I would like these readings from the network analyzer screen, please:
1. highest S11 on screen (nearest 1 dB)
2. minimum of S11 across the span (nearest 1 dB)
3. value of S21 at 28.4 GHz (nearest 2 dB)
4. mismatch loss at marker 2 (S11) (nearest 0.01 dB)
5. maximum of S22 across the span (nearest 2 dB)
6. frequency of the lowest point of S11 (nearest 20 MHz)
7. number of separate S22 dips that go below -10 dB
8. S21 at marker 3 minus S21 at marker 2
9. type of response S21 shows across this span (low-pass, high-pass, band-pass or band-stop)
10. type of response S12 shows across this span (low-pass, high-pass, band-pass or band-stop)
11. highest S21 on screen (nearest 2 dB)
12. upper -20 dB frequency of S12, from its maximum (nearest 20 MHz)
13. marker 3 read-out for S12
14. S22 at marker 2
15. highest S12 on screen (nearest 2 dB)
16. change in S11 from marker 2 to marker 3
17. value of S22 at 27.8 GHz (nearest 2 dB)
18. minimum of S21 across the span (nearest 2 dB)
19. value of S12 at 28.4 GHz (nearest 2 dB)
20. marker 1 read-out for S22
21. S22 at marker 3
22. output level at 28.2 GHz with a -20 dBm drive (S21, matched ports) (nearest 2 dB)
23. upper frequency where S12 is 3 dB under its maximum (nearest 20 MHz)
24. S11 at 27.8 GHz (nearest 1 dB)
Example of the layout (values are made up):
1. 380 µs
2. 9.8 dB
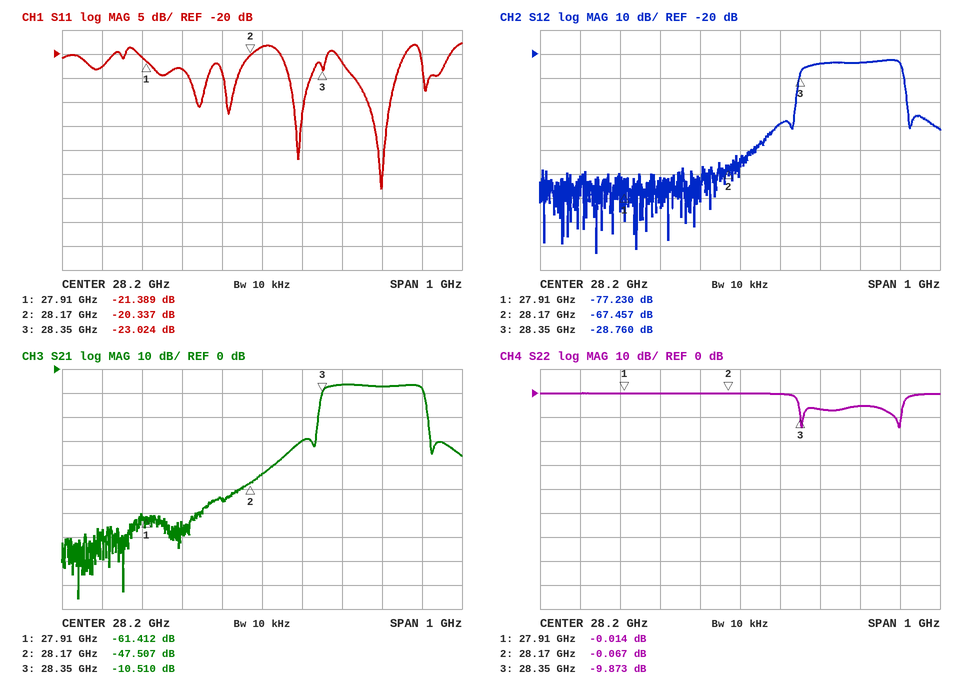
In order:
1. -18 dB
2. -48 dB
3. -6 dB
4. 0.04 dB
5. 0 dB
6. 28.50 GHz
7. 2
8. 36.997 dB
9. band-pass
10. band-pass
11. -6 dB
12. 28.62 GHz
13. -28.760 dB
14. -0.067 dB
15. -22 dB
16. -2.687 dB
17. 0 dB
18. -96 dB
19. -24 dB
20. -0.014 dB
21. -9.873 dB
22. -64 dBm
23. 28.60 GHz
24. -23 dB
